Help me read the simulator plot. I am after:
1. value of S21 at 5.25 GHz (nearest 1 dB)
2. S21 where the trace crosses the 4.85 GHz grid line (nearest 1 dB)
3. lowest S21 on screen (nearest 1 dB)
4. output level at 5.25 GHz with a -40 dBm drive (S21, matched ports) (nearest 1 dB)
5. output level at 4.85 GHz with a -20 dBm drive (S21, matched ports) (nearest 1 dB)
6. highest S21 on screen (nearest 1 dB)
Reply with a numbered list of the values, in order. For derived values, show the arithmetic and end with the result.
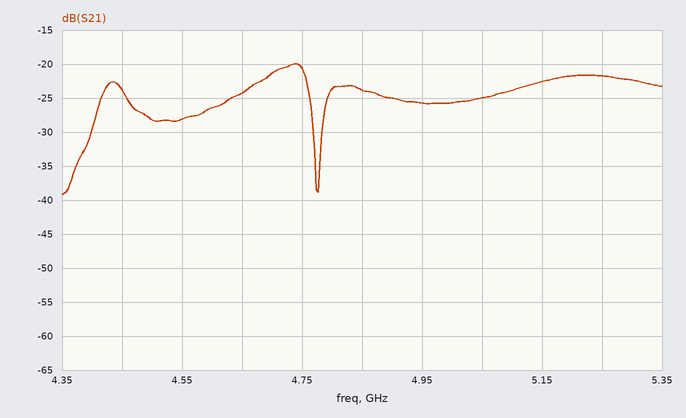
1. -22 dB
2. -24 dB
3. -39 dB
4. -40 dBm + (-22 dB) = -62 dBm
5. -20 dBm + (-24 dB) = -44 dBm
6. -20 dB
